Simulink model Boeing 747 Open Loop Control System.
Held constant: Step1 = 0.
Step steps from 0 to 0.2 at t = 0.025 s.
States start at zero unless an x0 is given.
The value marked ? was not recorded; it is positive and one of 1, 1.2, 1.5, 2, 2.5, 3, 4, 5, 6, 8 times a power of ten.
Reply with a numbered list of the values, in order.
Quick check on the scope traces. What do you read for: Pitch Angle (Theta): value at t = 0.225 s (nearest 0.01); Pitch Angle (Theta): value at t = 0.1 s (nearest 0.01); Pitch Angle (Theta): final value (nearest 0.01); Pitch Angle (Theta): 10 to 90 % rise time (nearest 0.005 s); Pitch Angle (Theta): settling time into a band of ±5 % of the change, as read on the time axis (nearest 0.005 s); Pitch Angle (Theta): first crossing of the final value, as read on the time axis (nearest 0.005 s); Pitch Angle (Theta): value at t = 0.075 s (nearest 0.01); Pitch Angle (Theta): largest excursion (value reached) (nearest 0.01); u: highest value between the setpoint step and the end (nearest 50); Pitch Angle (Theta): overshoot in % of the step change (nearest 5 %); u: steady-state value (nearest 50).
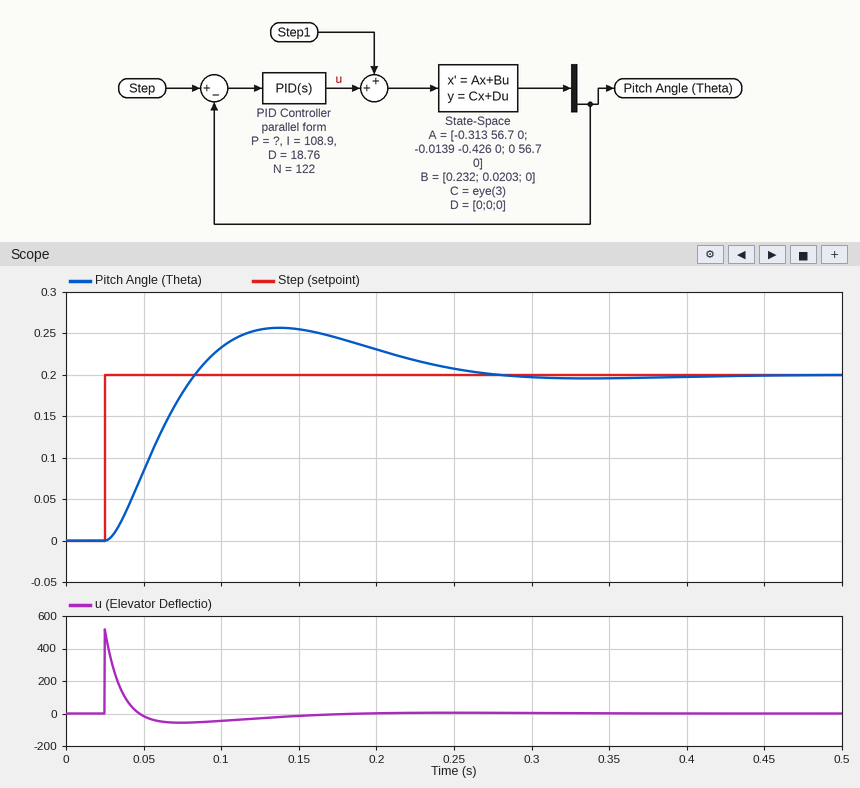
1. 0.22
2. 0.23
3. 0.20
4. 0.040 s
5. 0.245 s
6. 0.085 s
7. 0.18
8. 0.26
9. 500
10. 30 %
11. 0
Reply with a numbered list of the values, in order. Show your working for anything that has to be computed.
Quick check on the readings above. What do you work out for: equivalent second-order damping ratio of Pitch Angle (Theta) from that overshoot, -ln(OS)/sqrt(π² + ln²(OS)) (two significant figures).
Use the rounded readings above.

1. ln(0.3) = -1.204; 1.204 / sqrt(9.870 + 1.450) = 0.36
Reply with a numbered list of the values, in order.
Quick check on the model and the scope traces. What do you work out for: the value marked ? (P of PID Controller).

1. 300
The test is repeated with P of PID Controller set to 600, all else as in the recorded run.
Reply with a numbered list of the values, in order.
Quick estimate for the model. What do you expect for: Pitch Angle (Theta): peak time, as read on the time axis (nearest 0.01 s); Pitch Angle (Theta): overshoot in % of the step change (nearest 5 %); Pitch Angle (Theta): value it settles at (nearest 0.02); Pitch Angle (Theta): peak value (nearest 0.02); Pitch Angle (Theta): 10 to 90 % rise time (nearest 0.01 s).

1. 0.11 s
2. 40 %
3. 0.20
4. 0.28
5. 0.03 s
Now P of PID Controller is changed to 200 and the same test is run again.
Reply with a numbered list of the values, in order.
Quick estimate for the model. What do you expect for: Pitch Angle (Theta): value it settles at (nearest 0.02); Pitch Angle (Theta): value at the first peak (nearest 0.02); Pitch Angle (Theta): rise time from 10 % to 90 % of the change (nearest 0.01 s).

1. 0.20
2. 0.24
3. 0.05 s
